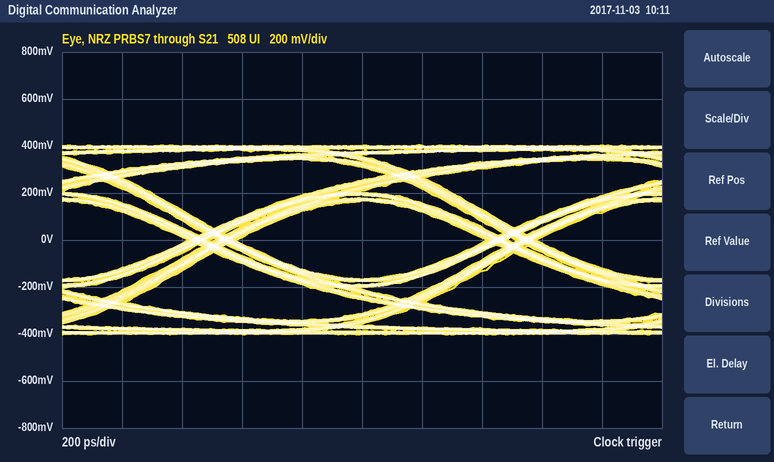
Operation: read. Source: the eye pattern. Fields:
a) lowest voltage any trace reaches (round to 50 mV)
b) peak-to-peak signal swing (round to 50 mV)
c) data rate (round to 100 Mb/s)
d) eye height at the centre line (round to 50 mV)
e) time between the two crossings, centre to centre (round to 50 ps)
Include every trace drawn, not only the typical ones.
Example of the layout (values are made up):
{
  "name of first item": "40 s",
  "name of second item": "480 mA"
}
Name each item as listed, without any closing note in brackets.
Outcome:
{
  "lowest voltage any trace reaches": "-400 mV",
  "peak-to-peak signal swing": "800 mV",
  "data rate": "1.0 Gb/s",
  "eye height at the centre line": "350 mV",
  "time between the two crossings, centre to centre": "1.00 ns"
}
